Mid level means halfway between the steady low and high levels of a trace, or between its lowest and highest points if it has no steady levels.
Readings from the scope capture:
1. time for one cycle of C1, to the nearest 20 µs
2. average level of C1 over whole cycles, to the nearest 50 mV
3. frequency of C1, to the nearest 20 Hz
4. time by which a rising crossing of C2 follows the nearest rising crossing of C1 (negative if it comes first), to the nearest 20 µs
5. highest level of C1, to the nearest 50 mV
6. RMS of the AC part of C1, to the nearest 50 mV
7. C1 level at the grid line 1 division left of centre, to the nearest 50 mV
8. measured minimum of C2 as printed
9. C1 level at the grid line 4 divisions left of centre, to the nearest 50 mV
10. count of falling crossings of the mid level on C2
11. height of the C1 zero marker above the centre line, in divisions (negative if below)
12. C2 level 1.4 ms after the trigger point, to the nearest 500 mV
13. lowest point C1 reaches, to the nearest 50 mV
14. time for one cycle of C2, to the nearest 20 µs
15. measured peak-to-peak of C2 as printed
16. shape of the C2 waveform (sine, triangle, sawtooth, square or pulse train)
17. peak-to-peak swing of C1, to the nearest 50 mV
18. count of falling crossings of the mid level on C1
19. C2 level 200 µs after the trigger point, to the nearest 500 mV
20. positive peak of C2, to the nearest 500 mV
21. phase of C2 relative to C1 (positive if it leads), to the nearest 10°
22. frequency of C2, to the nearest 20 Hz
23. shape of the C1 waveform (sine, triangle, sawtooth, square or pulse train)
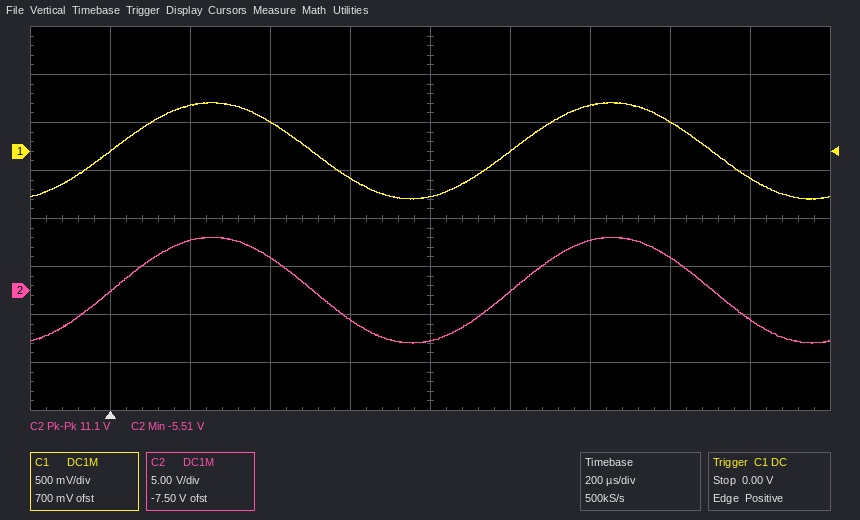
1.00 ms
0 mV
1.00 kHz
0 µs
500 mV
350 mV
-300 mV
-5.51 V
0 mV
2
+1.4 div
3.5 V
-500 mV
1.00 ms
11.1 V
sine
1.00 V
2
5.0 V
5.5 V
0°
1.00 kHz
sine
